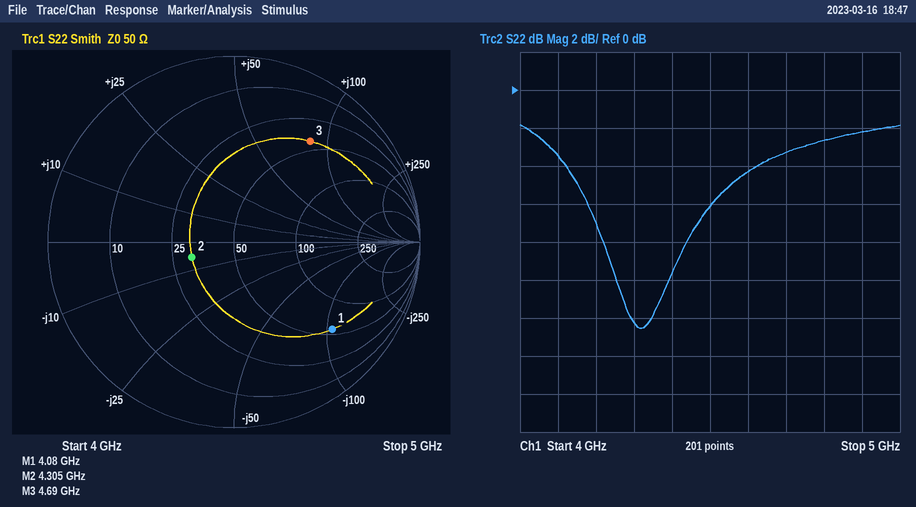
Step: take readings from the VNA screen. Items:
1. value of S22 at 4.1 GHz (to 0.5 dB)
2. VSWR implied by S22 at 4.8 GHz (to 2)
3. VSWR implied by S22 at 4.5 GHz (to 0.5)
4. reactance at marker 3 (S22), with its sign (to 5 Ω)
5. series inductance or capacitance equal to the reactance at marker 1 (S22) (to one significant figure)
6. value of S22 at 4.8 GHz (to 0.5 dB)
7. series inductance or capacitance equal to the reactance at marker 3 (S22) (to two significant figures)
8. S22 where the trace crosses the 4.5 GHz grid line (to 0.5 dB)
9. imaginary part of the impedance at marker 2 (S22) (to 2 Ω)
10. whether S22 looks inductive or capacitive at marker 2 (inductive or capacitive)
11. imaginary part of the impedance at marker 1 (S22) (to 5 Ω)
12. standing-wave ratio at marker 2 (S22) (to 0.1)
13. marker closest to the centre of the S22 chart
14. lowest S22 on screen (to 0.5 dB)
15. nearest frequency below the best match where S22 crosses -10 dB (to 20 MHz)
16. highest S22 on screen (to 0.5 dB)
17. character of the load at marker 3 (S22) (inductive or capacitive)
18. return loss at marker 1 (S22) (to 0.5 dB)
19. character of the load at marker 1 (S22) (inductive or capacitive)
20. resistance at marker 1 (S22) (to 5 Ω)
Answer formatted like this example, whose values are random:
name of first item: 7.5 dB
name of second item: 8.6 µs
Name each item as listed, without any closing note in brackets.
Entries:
value of S22 at 4.1 GHz: -3.5 dB
VSWR implied by S22 at 4.8 GHz: 6
VSWR implied by S22 at 4.5 GHz: 3.0
reactance at marker 3 (S22), with its sign: +85 Ω
series inductance or capacitance equal to the reactance at marker 1 (S22): 400 fF
value of S22 at 4.8 GHz: -2.5 dB
series inductance or capacitance equal to the reactance at marker 3 (S22): 2.9 nH
S22 where the trace crosses the 4.5 GHz grid line: -6.0 dB
imaginary part of the impedance at marker 2 (S22): -6 Ω
whether S22 looks inductive or capacitive at marker 2: capacitive
imaginary part of the impedance at marker 1 (S22): -105 Ω
standing-wave ratio at marker 2 (S22): 1.6
marker closest to the centre of the S22 chart: marker 2
lowest S22 on screen: -12.5 dB
nearest frequency below the best match where S22 crosses -10 dB: 4.26 GHz
highest S22 on screen: -2.0 dB
character of the load at marker 3 (S22): inductive
return loss at marker 1 (S22): 3.0 dB
character of the load at marker 1 (S22): capacitive
resistance at marker 1 (S22): 55 Ω
